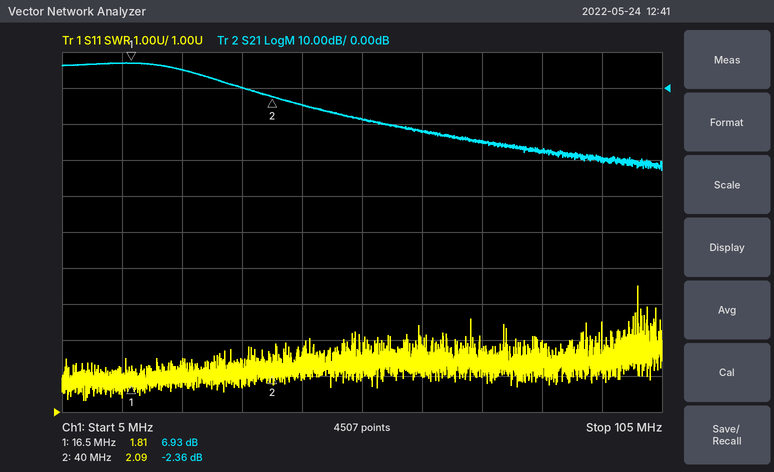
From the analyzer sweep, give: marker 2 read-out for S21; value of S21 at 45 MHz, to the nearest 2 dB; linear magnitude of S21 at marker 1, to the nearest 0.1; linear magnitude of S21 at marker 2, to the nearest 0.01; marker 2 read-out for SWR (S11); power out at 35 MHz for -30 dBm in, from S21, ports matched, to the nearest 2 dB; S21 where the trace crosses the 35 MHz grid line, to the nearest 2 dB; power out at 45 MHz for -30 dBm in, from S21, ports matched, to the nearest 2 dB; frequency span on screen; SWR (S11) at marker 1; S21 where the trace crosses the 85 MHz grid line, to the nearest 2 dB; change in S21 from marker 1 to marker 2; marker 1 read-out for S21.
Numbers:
-2.36 dB
-4 dB
2.2
0.76
2.09
-30 dBm
0 dB
-34 dBm
100 MHz
1.81
-18 dB
-9.29 dB
6.93 dB
